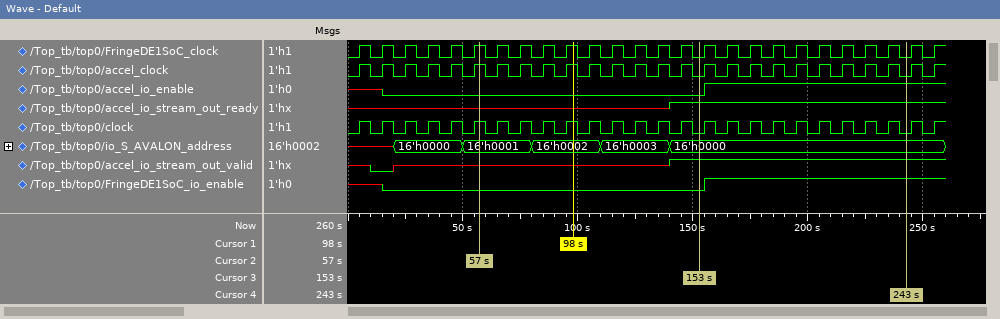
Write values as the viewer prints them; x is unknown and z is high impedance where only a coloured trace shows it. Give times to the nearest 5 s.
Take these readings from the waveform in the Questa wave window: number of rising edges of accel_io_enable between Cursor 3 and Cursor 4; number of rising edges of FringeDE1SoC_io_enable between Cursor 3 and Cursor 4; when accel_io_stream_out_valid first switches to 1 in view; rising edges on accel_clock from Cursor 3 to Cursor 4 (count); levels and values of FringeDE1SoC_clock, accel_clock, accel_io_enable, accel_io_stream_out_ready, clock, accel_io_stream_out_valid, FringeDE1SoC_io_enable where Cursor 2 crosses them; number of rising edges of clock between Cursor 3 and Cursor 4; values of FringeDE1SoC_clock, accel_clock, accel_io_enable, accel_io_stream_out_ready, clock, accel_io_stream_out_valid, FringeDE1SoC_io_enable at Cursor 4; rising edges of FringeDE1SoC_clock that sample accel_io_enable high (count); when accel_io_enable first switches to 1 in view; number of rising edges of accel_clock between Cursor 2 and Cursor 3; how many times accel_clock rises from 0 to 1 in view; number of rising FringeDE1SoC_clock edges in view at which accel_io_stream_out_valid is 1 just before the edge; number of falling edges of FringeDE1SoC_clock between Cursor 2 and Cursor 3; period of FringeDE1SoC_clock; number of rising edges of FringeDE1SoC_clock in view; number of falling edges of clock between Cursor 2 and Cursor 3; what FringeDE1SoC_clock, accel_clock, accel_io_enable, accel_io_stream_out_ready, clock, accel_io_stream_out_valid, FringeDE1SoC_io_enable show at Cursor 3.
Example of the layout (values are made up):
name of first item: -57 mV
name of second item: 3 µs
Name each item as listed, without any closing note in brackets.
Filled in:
number of rising edges of accel_io_enable between Cursor 3 and Cursor 4: 1
number of rising edges of FringeDE1SoC_io_enable between Cursor 3 and Cursor 4: 1
when accel_io_stream_out_valid first switches to 1 in view: 140 s
rising edges on accel_clock from Cursor 3 to Cursor 4: 9
levels and values of FringeDE1SoC_clock, accel_clock, accel_io_enable, accel_io_stream_out_ready, clock, accel_io_stream_out_valid, FringeDE1SoC_io_enable where Cursor 2 crosses them: FringeDE1SoC_clock=1, accel_clock=1, accel_io_enable=0, accel_io_stream_out_ready=x, clock=1, accel_io_stream_out_valid=x, FringeDE1SoC_io_enable=0
number of rising edges of clock between Cursor 3 and Cursor 4: 9
values of FringeDE1SoC_clock, accel_clock, accel_io_enable, accel_io_stream_out_ready, clock, accel_io_stream_out_valid, FringeDE1SoC_io_enable at Cursor 4: FringeDE1SoC_clock=0, accel_clock=0, accel_io_enable=1, accel_io_stream_out_ready=1, clock=0, accel_io_stream_out_valid=1, FringeDE1SoC_io_enable=1
rising edges of FringeDE1SoC_clock that sample accel_io_enable high: 10
when accel_io_enable first switches to 1 in view: 155 s
number of rising edges of accel_clock between Cursor 2 and Cursor 3: 9
how many times accel_clock rises from 0 to 1 in view: 26
number of rising FringeDE1SoC_clock edges in view at which accel_io_stream_out_valid is 1 just before the edge: 12
number of falling edges of FringeDE1SoC_clock between Cursor 2 and Cursor 3: 10
period of FringeDE1SoC_clock: 10 s
number of rising edges of FringeDE1SoC_clock in view: 26
number of falling edges of clock between Cursor 2 and Cursor 3: 10
what FringeDE1SoC_clock, accel_clock, accel_io_enable, accel_io_stream_out_ready, clock, accel_io_stream_out_valid, FringeDE1SoC_io_enable show at Cursor 3: FringeDE1SoC_clock=0, accel_clock=0, accel_io_enable=0, accel_io_stream_out_ready=1, clock=0, accel_io_stream_out_valid=1, FringeDE1SoC_io_enable=0
